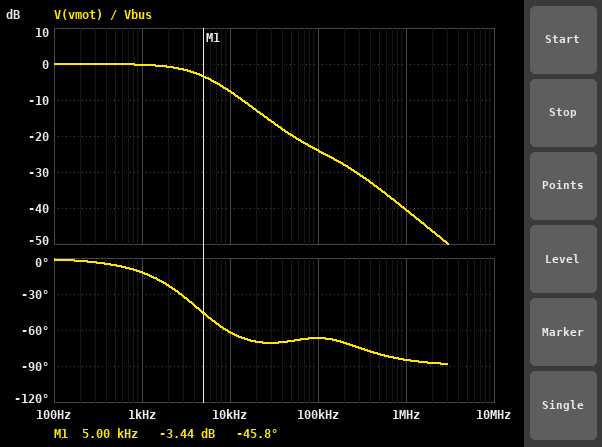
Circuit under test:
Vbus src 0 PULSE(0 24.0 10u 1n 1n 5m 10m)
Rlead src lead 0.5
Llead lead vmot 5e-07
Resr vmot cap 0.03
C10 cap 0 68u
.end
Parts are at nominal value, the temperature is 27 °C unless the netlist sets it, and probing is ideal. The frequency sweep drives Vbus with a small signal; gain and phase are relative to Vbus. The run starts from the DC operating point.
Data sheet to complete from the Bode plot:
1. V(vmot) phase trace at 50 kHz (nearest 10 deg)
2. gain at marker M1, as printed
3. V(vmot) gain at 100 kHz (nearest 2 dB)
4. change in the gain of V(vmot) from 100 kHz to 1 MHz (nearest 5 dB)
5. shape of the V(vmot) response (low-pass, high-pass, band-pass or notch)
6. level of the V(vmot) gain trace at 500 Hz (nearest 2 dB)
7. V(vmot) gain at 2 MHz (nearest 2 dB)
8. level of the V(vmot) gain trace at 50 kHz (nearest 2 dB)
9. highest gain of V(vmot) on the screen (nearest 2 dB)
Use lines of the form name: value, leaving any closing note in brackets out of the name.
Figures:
V(vmot) phase trace at 50 kHz: -70 deg
gain at marker M1, as printed: -3.44 dB
V(vmot) gain at 100 kHz: -24 dB
change in the gain of V(vmot) from 100 kHz to 1 MHz: -15 dB
shape of the V(vmot) response: low-pass
level of the V(vmot) gain trace at 500 Hz: 0 dB
V(vmot) gain at 2 MHz: -46 dB
level of the V(vmot) gain trace at 50 kHz: -20 dB
highest gain of V(vmot) on the screen: 0 dB
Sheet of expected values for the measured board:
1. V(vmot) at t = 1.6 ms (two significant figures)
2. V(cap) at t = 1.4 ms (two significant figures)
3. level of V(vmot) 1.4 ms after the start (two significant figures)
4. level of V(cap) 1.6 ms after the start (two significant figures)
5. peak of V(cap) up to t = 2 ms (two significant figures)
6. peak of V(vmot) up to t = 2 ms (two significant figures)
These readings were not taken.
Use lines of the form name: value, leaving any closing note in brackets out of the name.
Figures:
V(vmot) at t = 1.6 ms: 24 V
V(cap) at t = 1.4 ms: 24 V
level of V(vmot) 1.4 ms after the start: 24 V
level of V(cap) 1.6 ms after the start: 24 V
peak of V(cap) up to t = 2 ms: 24 V
peak of V(vmot) up to t = 2 ms: 24 V
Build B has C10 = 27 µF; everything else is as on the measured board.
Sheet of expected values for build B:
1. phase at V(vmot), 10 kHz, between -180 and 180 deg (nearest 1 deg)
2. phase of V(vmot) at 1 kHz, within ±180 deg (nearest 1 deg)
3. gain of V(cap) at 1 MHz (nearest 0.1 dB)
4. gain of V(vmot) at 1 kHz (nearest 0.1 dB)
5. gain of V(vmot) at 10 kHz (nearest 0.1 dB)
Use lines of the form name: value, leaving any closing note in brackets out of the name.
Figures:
phase at V(vmot), 10 kHz, between -180 and 180 deg: -41 deg
phase of V(vmot) at 1 kHz, within ±180 deg: -5 deg
gain of V(cap) at 1 MHz: -54.6 dB
gain of V(vmot) at 1 kHz: 0 dB
gain of V(vmot) at 10 kHz: -2.3 dB
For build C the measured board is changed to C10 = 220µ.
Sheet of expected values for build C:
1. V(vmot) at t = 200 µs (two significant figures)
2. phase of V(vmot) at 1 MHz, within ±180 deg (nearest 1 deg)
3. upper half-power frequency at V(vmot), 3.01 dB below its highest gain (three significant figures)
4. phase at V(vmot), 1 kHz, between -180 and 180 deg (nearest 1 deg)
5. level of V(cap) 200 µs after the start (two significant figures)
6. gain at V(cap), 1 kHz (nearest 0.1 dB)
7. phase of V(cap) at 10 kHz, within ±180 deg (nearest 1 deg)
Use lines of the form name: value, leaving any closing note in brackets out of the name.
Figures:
V(vmot) at t = 200 µs: 20 V
phase of V(vmot) at 1 MHz, within ±180 deg: -82 deg
upper half-power frequency at V(vmot), 3.01 dB below its highest gain: 1.38 kHz
phase at V(vmot), 1 kHz, between -180 and 180 deg: -34 deg
level of V(cap) 200 µs after the start: 19 V
gain at V(cap), 1 kHz: -1.8 dB
phase of V(cap) at 10 kHz, within ±180 deg: -86 deg
